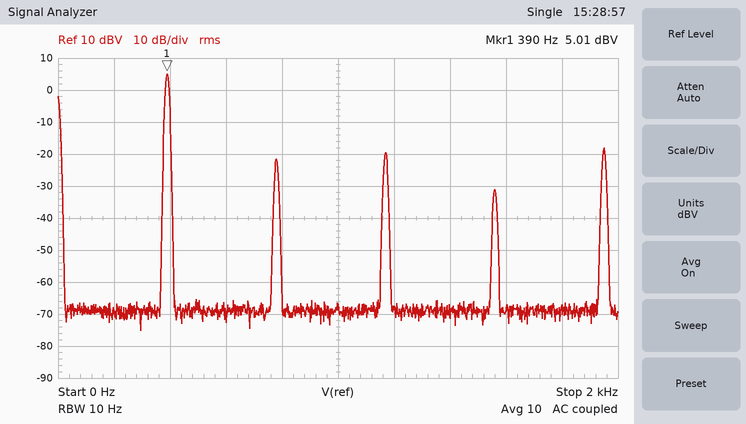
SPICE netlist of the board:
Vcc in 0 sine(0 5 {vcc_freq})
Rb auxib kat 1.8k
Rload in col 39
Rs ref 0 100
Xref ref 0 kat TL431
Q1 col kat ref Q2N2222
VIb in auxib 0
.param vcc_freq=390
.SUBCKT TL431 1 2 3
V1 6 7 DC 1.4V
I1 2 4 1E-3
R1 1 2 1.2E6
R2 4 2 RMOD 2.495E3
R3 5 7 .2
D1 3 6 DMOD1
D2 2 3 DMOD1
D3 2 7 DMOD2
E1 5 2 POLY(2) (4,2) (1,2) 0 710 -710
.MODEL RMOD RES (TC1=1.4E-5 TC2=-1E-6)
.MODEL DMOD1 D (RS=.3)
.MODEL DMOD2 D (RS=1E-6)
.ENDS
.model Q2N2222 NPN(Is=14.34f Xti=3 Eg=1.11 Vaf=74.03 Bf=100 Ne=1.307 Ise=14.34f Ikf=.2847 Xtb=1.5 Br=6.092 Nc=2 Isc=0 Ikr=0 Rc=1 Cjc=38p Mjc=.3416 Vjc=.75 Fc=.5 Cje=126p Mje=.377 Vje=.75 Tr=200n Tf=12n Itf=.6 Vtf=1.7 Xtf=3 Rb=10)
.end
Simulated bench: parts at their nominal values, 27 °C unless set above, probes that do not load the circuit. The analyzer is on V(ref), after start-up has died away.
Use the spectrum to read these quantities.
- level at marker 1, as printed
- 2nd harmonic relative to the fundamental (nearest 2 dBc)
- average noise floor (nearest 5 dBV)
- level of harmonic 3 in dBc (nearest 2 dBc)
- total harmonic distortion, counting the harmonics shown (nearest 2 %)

5.01 dBV
-26 dBc
-70 dBV
-24 dBc
10 %
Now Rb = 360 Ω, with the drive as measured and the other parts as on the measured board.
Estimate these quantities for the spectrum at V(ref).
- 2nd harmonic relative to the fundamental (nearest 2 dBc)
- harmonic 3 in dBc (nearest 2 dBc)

-30 dBc
-22 dBc
